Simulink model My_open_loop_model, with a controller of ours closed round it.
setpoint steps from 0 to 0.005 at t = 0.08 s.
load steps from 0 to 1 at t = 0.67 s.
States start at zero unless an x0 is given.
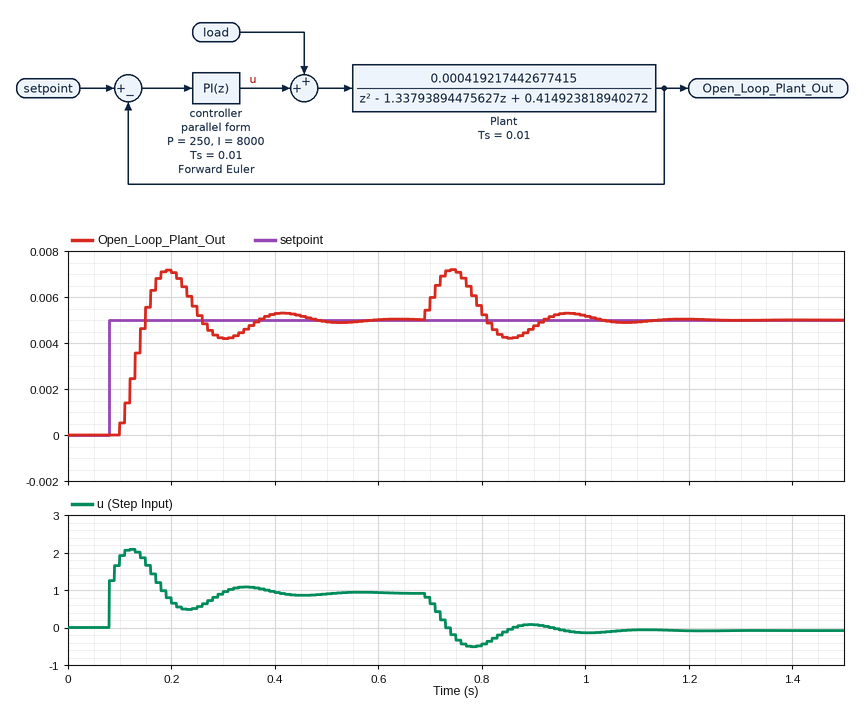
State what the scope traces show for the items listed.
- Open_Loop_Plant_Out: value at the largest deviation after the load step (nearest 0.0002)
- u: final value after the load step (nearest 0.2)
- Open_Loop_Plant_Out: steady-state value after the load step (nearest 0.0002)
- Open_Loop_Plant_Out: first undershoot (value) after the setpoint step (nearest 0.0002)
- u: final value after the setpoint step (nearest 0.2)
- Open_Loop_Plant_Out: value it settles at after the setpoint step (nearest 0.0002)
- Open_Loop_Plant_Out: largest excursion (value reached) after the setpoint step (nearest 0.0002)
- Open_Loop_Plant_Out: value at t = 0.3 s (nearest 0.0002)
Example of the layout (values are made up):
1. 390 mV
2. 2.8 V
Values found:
1. 0.0072
2. 0.0
3. 0.0050
4. 0.0042
5. 1.0
6. 0.0050
7. 0.0072
8. 0.0042
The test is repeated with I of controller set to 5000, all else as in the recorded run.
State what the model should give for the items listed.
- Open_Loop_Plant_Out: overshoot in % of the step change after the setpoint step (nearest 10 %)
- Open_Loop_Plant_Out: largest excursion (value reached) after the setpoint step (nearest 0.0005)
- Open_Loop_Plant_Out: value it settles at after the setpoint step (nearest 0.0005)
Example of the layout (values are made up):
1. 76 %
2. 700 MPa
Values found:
1. 20 %
2. 0.0060
3. 0.0050
